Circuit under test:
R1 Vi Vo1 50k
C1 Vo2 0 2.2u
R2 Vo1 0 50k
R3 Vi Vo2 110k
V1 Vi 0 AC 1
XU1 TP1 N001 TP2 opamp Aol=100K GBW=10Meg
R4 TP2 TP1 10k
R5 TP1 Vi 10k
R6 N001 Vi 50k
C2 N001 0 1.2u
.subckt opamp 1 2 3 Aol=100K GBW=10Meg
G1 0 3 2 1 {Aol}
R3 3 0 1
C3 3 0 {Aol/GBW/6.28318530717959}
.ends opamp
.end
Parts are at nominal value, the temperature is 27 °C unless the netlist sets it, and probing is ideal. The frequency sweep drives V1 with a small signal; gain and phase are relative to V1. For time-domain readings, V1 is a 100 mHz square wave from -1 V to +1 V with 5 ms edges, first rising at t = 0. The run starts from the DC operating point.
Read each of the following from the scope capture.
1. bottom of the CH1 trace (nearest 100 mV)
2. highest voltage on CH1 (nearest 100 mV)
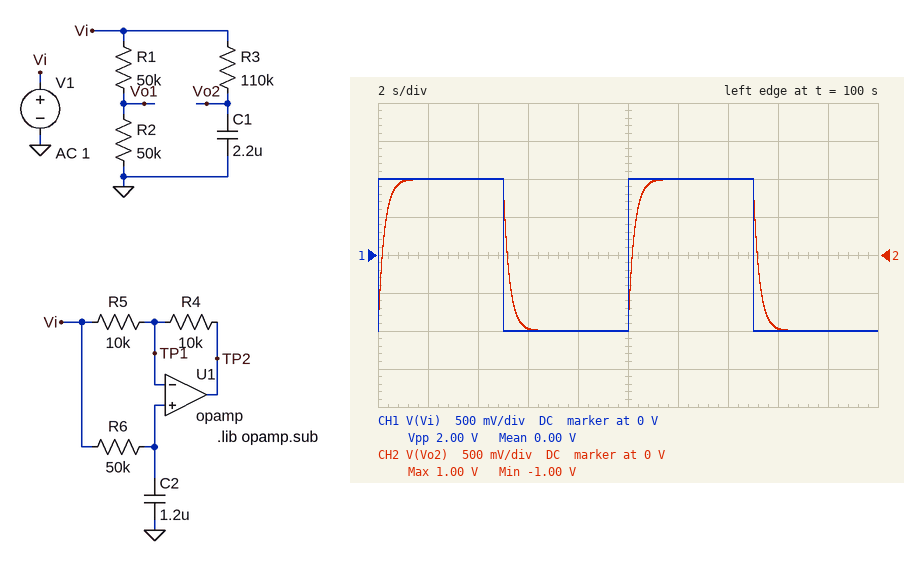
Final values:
-1.0 V
1.0 V
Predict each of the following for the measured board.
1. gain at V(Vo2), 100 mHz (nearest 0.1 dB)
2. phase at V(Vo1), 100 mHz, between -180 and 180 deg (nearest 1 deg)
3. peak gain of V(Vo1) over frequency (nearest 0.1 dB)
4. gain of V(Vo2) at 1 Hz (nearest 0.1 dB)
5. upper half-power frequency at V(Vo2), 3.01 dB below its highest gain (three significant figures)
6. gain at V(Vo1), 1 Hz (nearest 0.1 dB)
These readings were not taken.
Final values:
-0.1 dB
0 deg
-6.0 dB
-5.2 dB
658 mHz
-6.0 dB
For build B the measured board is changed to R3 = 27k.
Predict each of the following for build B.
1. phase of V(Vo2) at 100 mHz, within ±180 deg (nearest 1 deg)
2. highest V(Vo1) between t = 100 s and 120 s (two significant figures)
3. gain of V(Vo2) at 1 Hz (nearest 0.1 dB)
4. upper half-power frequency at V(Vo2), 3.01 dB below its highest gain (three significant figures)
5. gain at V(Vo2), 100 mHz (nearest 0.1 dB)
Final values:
-2 deg
500 mV
-0.6 dB
2.68 Hz
0 dB
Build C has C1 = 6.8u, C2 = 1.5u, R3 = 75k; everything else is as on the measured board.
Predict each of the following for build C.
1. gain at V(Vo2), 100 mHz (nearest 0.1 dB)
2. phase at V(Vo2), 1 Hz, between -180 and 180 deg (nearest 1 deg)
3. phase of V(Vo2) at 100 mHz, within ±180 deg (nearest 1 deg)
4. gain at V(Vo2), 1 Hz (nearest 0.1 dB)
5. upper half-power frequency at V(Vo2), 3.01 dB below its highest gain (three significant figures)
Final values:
-0.4 dB
-73 deg
-18 deg
-10.5 dB
312 mHz
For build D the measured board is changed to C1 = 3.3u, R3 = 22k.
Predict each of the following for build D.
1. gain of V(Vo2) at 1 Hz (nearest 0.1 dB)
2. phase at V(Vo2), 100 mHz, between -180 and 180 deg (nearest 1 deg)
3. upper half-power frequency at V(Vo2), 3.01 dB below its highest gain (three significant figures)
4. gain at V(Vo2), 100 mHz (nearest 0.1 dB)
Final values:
-0.8 dB
-3 deg
2.19 Hz
0 dB
